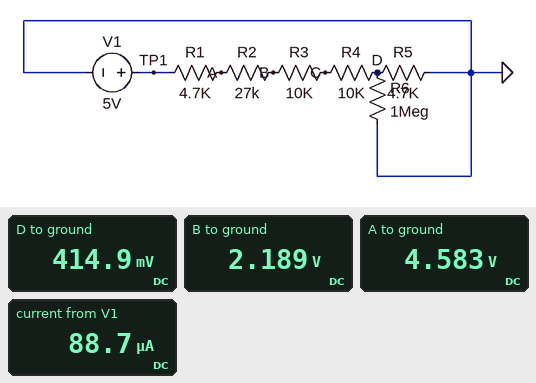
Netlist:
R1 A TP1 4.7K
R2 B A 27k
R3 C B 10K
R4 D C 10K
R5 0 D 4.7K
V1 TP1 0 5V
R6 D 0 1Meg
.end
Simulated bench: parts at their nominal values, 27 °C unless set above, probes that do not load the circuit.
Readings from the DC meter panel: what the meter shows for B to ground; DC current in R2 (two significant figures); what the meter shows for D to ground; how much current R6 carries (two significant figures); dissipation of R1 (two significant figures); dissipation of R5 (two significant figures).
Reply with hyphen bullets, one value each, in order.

- 2.189 V
- 89 µA
- 414.9 mV
- 410 nA
- 37 µW
- 37 µW
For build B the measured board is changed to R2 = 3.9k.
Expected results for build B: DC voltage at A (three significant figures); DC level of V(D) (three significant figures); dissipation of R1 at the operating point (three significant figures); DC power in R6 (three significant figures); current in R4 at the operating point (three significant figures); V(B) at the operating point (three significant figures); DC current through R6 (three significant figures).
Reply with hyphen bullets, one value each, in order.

- 4.29 V
- 703 mV
- 106 µW
- 494 nW
- 150 µA
- 3.71 V
- 703 nA
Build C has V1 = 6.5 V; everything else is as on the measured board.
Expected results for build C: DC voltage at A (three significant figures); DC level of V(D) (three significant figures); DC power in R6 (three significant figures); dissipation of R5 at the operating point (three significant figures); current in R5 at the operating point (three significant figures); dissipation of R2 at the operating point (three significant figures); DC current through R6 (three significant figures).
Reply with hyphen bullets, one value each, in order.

- 5.96 V
- 539 mV
- 291 nW
- 61.9 µW
- 115 µA
- 359 µW
- 539 nA
